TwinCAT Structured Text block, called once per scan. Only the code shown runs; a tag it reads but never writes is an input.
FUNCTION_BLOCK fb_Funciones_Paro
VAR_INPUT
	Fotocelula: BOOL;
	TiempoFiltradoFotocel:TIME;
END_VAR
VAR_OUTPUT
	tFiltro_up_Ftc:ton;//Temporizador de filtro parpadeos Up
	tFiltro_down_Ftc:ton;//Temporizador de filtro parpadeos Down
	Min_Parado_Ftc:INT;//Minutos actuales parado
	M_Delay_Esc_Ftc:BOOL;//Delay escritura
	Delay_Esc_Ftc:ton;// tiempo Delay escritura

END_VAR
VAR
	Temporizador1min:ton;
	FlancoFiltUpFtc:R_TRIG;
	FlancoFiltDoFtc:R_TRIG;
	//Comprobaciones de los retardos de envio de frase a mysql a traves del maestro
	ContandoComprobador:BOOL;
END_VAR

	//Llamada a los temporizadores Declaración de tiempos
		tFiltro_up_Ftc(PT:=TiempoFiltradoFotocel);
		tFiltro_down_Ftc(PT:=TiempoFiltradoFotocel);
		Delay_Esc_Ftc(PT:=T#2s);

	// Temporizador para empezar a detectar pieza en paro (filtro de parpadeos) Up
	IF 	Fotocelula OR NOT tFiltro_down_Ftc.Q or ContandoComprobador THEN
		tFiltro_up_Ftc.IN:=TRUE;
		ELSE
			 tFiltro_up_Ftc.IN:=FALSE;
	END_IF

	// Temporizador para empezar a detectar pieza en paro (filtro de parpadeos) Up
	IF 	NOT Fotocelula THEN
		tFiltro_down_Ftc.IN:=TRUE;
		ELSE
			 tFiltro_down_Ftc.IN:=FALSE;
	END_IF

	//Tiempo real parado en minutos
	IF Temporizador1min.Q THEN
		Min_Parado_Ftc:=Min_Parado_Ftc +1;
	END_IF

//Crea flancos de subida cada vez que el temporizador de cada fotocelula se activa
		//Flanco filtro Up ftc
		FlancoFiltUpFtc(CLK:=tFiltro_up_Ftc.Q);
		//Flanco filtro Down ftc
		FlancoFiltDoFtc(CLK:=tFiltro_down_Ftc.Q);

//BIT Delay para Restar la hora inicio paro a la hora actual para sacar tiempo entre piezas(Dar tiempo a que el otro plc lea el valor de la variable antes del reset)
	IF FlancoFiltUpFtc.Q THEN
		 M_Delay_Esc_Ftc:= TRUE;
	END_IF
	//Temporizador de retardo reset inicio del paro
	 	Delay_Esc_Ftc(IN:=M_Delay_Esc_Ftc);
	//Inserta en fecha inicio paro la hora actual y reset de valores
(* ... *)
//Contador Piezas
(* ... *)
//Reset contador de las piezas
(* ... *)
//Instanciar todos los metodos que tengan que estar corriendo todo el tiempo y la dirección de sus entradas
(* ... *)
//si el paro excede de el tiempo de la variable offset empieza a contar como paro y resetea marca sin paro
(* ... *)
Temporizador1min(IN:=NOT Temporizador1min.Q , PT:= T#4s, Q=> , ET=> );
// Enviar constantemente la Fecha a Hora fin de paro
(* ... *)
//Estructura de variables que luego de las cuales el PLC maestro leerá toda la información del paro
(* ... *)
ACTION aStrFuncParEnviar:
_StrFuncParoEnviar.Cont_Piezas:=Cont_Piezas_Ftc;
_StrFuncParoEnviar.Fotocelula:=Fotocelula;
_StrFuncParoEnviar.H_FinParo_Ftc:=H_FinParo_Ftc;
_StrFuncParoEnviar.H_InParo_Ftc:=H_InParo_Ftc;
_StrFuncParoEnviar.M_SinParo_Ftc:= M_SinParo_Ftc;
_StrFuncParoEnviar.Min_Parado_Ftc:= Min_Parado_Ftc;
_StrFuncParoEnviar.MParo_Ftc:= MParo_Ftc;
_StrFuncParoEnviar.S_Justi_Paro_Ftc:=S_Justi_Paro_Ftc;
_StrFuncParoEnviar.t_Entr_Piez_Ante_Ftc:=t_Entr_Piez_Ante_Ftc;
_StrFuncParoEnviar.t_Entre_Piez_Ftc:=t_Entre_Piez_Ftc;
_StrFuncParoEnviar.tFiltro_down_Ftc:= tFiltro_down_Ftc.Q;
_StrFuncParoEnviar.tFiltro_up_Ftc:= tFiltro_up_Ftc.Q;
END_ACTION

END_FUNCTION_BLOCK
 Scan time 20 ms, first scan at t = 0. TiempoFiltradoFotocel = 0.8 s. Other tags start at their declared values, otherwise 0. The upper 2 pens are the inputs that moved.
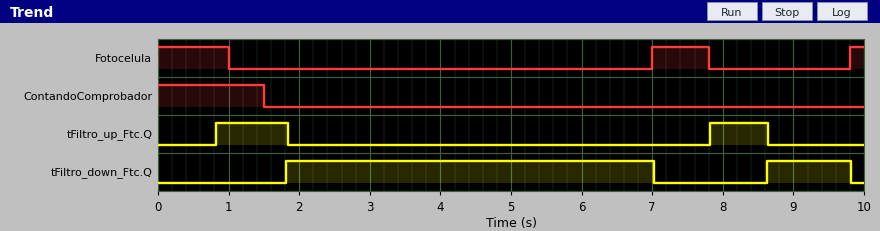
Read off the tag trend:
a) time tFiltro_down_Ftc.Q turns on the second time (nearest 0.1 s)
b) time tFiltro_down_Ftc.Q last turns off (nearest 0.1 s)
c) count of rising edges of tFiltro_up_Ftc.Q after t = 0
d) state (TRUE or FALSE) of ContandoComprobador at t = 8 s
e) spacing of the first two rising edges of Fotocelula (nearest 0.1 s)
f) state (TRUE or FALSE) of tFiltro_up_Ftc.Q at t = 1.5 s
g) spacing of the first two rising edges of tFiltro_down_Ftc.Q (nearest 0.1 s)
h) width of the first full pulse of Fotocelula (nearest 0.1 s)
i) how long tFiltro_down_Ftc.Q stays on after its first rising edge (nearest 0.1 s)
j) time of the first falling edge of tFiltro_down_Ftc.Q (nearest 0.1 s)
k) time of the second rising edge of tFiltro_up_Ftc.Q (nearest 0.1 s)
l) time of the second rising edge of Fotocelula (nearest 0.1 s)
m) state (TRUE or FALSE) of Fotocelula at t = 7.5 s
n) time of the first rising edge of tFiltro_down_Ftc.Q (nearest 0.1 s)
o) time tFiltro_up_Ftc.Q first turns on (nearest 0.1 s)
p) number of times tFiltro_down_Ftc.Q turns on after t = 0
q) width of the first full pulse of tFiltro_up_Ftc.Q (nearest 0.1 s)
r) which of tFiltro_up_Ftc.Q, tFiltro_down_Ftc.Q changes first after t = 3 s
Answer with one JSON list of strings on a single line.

["8.6 s", "9.8 s", "2", "FALSE", "2.8 s", "TRUE", "6.8 s", "0.8 s", "5.2 s", "7.0 s", "7.8 s", "9.8 s", "TRUE", "1.8 s", "0.8 s", "2", "1.0 s", "tFiltro_down_Ftc.Q"]
